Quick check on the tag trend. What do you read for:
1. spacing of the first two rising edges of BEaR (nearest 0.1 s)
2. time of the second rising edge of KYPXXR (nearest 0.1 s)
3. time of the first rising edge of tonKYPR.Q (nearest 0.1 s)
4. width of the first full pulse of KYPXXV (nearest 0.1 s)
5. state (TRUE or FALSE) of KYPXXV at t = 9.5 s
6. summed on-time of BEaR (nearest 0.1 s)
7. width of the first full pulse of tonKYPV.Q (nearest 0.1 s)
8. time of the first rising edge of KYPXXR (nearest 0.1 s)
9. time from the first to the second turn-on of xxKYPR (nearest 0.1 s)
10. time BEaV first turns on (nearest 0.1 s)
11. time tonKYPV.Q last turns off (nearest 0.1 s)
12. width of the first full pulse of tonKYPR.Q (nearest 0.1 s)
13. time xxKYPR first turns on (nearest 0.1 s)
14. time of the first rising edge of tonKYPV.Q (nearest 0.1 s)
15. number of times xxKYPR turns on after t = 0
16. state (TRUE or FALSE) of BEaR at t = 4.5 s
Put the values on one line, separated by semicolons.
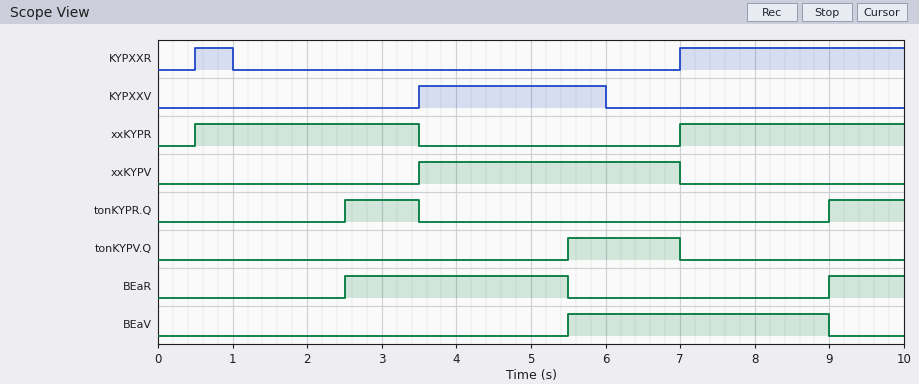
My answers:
6.5 s; 7.0 s; 2.5 s; 2.5 s; FALSE; 4.0 s; 1.5 s; 0.5 s; 6.5 s; 5.5 s; 7.0 s; 1.0 s; 0.5 s; 5.5 s; 2; TRUE
